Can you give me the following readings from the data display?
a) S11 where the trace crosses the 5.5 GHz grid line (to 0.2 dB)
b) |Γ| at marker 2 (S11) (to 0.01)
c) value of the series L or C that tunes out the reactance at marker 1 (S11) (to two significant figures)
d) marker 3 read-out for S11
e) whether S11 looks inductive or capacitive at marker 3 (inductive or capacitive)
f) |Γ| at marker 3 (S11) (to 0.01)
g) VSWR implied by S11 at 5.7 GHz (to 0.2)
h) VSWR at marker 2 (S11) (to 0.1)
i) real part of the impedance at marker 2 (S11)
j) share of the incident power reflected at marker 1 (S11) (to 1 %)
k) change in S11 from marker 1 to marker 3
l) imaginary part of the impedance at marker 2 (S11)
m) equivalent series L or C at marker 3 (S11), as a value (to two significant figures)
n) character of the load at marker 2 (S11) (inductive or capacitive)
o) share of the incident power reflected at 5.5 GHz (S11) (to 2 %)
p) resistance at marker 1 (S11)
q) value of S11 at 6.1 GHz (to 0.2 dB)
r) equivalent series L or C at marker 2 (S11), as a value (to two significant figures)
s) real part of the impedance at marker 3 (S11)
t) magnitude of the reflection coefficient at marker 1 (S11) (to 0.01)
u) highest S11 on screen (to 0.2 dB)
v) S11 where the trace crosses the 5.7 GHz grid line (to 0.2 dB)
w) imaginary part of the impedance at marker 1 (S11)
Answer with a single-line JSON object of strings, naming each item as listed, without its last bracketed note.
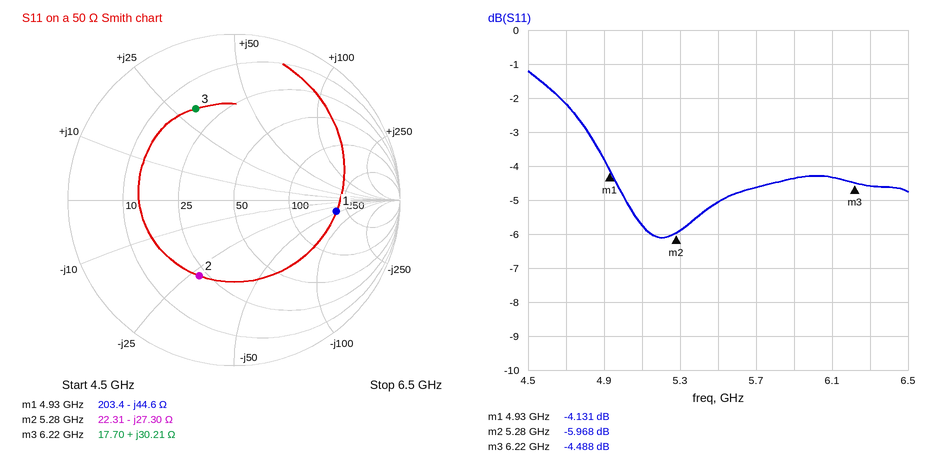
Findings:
{"S11 where the trace crosses the 5.5 GHz grid line": "-5.0 dB", "|Γ| at marker 2 (S11)": "0.50", "value of the series L or C that tunes out the reactance at marker 1 (S11)": "1.4 nH", "marker 3 read-out for S11": "-4.488 dB", "whether S11 looks inductive or capacitive at marker 3": "inductive", "|Γ| at marker 3 (S11)": "0.60", "VSWR implied by S11 at 5.7 GHz": "3.8", "VSWR at marker 2 (S11)": "3.0", "real part of the impedance at marker 2": "22.31 Ω", "share of the incident power reflected at marker 1 (S11)": "39 %", "change in S11 from marker 1 to marker 3": "-0.357 dB", "imaginary part of the impedance at marker 2": "-27.30 Ω", "equivalent series L or C at marker 3 (S11), as a value": "770 pH", "character of the load at marker 2 (S11)": "capacitive", "share of the incident power reflected at 5.5 GHz (S11)": "32 %", "resistance at marker 1": "203.4 Ω", "value of S11 at 6.1 GHz": "-4.4 dB", "equivalent series L or C at marker 2 (S11), as a value": "1.1 pF", "real part of the impedance at marker 3": "17.70 Ω", "magnitude of the reflection coefficient at marker 1 (S11)": "0.62", "highest S11 on screen": "-1.2 dB", "S11 where the trace crosses the 5.7 GHz grid line": "-4.6 dB", "imaginary part of the impedance at marker 1": "-44.6 Ω"}
